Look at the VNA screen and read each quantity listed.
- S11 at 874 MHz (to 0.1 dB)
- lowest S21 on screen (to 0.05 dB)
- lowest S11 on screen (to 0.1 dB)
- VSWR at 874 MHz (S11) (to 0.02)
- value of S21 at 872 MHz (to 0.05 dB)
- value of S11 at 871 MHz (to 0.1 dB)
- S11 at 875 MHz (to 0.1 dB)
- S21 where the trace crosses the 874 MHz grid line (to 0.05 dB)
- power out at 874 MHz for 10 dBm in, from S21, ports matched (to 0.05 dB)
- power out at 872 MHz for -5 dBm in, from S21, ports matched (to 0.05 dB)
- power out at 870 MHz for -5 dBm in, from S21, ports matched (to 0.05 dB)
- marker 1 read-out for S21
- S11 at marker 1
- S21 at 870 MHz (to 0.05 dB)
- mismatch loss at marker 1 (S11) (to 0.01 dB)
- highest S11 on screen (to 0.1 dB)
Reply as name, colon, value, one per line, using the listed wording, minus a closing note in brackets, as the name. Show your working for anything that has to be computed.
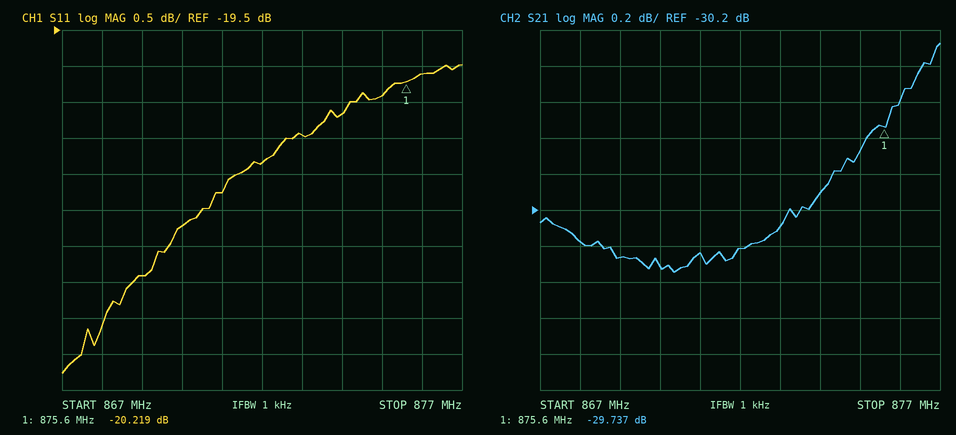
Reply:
S11 at 874 MHz: -20.7 dB
lowest S21 on screen: -30.55 dB
lowest S11 on screen: -24.3 dB
VSWR at 874 MHz (S11): |Γ| = 10^(-20.7/20) = 0.0923; VSWR = (1 + 0.0923)/(1 − 0.0923) ≈ 1.20
value of S21 at 872 MHz: -30.40 dB
value of S11 at 871 MHz: -21.8 dB
S11 at 875 MHz: -20.4 dB
S21 where the trace crosses the 874 MHz grid line: -30.10 dB
power out at 874 MHz for 10 dBm in, from S21, ports matched: 10 dBm + (-30.10 dB) = -20.10 dBm
power out at 872 MHz for -5 dBm in, from S21, ports matched: -5 dBm + (-30.40 dB) = -35.40 dBm
power out at 870 MHz for -5 dBm in, from S21, ports matched: -5 dBm + (-30.50 dB) = -35.50 dBm
marker 1 read-out for S21: -29.737 dB
S11 at marker 1: -20.219 dB
S21 at 870 MHz: -30.50 dB
mismatch loss at marker 1 (S11): −10 log10(1 − 10^(-20.219/10)) ≈ 0.04 dB
highest S11 on screen: -20.0 dB
